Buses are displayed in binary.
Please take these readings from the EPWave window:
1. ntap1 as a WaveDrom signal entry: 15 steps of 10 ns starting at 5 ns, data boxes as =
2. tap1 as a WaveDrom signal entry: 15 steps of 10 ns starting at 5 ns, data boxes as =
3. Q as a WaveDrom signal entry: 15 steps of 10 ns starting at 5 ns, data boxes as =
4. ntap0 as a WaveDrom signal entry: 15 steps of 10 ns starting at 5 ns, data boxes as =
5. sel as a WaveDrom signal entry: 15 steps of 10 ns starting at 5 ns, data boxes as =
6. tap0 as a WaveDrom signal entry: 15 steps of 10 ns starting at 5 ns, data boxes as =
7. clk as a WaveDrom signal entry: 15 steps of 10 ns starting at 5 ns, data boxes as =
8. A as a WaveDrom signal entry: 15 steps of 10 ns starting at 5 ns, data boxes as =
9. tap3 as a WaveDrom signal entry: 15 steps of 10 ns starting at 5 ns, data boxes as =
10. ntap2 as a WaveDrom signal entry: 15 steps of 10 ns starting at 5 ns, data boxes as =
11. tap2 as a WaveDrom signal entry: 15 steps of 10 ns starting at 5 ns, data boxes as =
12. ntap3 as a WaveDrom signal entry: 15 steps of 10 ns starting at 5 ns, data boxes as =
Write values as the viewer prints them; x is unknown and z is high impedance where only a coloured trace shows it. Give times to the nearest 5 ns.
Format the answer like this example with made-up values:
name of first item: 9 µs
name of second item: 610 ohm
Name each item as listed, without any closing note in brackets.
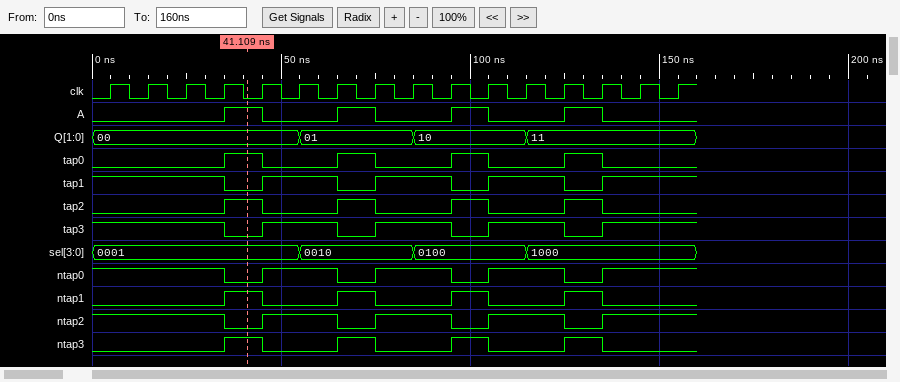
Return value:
ntap1 as a WaveDrom signal entry: 15 steps of 10 ns starting at 5 ns, data boxes as =: {name: 'ntap1', wave: '0..10.10.10.10.'}
tap1 as a WaveDrom signal entry: 15 steps of 10 ns starting at 5 ns, data boxes as =: {name: 'tap1', wave: '1..01.01.01.01.'}
Q as a WaveDrom signal entry: 15 steps of 10 ns starting at 5 ns, data boxes as =: {name: 'Q', wave: '=....=..=..=...', data: '00 01 10 11'}
ntap0 as a WaveDrom signal entry: 15 steps of 10 ns starting at 5 ns, data boxes as =: {name: 'ntap0', wave: '1..01.01.01.01.'}
sel as a WaveDrom signal entry: 15 steps of 10 ns starting at 5 ns, data boxes as =: {name: 'sel', wave: '=....=..=..=...', data: '0001 0010 0100 1000'}
tap0 as a WaveDrom signal entry: 15 steps of 10 ns starting at 5 ns, data boxes as =: {name: 'tap0', wave: '0..10.10.10.10.'}
clk as a WaveDrom signal entry: 15 steps of 10 ns starting at 5 ns, data boxes as =: {name: 'clk', wave: 'p..............'}
A as a WaveDrom signal entry: 15 steps of 10 ns starting at 5 ns, data boxes as =: {name: 'A', wave: '0..10.10.10.10.'}
tap3 as a WaveDrom signal entry: 15 steps of 10 ns starting at 5 ns, data boxes as =: {name: 'tap3', wave: '1..01.01.01.01.'}
ntap2 as a WaveDrom signal entry: 15 steps of 10 ns starting at 5 ns, data boxes as =: {name: 'ntap2', wave: '1..01.01.01.01.'}
tap2 as a WaveDrom signal entry: 15 steps of 10 ns starting at 5 ns, data boxes as =: {name: 'tap2', wave: '0..10.10.10.10.'}
ntap3 as a WaveDrom signal entry: 15 steps of 10 ns starting at 5 ns, data boxes as =: {name: 'ntap3', wave: '0..10.10.10.10.'}
